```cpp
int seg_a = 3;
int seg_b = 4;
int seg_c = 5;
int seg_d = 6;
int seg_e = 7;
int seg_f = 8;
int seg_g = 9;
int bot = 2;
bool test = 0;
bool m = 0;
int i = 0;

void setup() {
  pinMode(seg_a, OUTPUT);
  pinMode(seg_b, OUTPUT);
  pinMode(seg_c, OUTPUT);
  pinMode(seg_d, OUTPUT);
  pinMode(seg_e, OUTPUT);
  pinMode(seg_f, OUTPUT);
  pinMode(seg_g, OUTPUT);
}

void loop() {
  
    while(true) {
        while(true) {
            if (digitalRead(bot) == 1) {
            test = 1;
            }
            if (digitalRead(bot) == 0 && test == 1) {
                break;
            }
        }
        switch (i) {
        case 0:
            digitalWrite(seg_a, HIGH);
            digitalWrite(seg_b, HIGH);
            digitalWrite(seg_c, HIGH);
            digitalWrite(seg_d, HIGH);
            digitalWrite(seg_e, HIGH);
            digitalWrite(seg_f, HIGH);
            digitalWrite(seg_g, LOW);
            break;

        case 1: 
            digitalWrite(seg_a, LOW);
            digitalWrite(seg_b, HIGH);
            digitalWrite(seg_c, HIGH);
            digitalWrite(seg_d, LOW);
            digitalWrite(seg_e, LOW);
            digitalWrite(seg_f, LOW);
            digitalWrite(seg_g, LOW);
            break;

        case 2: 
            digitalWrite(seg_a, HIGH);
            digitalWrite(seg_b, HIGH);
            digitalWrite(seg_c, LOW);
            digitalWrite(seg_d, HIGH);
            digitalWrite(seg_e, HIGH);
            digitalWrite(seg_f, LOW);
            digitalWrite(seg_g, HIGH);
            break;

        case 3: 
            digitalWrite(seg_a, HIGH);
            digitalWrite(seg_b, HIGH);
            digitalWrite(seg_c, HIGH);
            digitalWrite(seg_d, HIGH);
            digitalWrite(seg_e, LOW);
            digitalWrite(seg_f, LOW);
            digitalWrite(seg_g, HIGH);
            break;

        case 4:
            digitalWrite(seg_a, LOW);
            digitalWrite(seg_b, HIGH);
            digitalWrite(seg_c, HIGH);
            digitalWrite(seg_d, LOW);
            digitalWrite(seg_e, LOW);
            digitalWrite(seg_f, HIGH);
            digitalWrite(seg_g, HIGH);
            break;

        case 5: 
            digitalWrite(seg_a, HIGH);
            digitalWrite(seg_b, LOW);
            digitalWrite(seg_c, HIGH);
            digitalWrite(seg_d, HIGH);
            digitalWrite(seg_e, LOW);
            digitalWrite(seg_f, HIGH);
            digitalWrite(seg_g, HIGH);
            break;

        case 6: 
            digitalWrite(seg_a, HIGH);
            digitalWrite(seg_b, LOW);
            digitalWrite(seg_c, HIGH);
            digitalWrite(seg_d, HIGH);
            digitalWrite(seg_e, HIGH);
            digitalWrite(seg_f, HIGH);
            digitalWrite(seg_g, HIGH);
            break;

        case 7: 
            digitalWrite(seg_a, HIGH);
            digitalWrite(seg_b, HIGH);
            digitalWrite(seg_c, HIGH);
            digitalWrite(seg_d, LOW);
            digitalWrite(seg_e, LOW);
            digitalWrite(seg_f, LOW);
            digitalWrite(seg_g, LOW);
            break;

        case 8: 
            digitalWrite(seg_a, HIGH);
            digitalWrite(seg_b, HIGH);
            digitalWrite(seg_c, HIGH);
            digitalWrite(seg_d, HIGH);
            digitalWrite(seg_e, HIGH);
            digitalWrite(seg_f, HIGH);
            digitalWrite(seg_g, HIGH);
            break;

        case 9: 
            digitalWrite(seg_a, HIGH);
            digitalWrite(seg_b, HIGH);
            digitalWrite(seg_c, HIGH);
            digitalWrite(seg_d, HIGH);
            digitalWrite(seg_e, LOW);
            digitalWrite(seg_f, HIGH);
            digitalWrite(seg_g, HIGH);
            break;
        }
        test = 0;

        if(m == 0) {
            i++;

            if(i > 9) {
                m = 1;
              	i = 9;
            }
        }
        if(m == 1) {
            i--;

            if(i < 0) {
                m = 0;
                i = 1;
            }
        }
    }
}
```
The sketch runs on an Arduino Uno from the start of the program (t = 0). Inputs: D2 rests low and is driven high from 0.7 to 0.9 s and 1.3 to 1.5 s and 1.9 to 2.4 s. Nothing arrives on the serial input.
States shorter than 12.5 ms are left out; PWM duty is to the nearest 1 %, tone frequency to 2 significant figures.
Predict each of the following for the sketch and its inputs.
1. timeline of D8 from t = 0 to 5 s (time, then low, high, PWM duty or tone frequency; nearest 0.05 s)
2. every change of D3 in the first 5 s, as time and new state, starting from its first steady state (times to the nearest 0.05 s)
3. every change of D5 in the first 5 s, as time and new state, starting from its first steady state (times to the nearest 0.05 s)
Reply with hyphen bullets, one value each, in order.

- 0 s low; 0.9 s high; 1.5 s low
- 0 s low; 0.9 s high; 1.5 s low; 2.4 s high
- 0 s low; 0.9 s high; 2.4 s low
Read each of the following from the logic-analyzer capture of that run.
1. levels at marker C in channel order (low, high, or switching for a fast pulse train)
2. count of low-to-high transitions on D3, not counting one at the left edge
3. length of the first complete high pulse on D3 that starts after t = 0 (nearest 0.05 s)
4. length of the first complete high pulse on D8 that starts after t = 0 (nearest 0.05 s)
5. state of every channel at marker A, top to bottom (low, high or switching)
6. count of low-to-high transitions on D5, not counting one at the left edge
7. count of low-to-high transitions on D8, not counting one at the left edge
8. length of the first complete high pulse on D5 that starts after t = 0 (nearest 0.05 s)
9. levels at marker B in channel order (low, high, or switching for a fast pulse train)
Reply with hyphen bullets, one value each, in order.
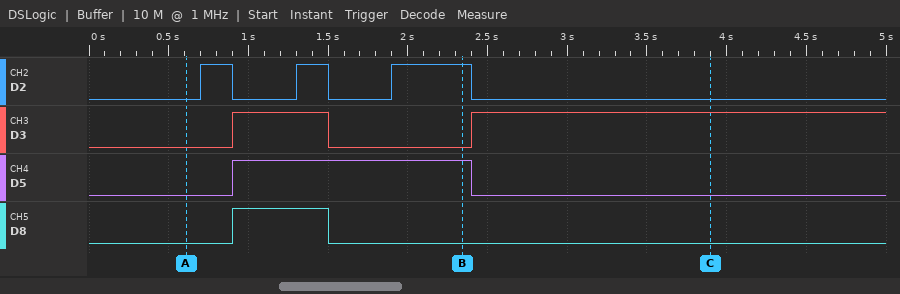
- D2 low, D3 high, D5 low, D8 low
- 2
- 0.60 s
- 0.60 s
- D2 low, D3 low, D5 low, D8 low
- 1
- 1
- 1.50 s
- D2 high, D3 low, D5 high, D8 low
